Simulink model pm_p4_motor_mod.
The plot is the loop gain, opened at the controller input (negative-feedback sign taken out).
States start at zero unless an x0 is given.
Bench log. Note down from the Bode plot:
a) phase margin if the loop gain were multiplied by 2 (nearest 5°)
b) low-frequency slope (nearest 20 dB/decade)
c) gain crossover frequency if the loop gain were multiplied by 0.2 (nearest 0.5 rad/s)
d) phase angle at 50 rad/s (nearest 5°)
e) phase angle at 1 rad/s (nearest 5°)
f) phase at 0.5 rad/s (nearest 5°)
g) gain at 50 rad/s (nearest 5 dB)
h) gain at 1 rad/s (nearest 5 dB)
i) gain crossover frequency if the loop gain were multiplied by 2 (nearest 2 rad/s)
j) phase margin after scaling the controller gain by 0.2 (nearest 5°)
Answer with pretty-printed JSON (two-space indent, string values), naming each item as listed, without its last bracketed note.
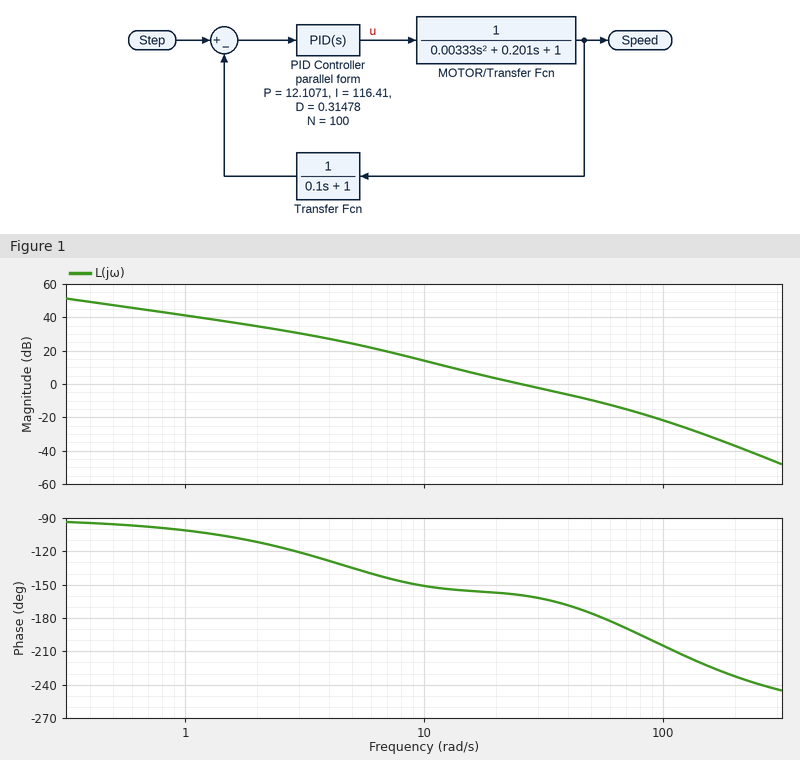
{
  "phase margin if the loop gain were multiplied by 2": "10°",
  "low-frequency slope": "-20 dB/decade",
  "gain crossover frequency if the loop gain were multiplied by 0.2": "10.0 rad/s",
  "phase angle at 50 rad/s": "-175°",
  "phase angle at 1 rad/s": "-100°",
  "phase at 0.5 rad/s": "-95°",
  "gain at 50 rad/s": "-10 dB",
  "gain at 1 rad/s": "40 dB",
  "gain crossover frequency if the loop gain were multiplied by 2": "40 rad/s",
  "phase margin after scaling the controller gain by 0.2": "30°"
}
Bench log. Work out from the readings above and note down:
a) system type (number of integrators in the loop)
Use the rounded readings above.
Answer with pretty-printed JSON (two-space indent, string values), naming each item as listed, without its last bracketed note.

{
  "system type": "1"
}
